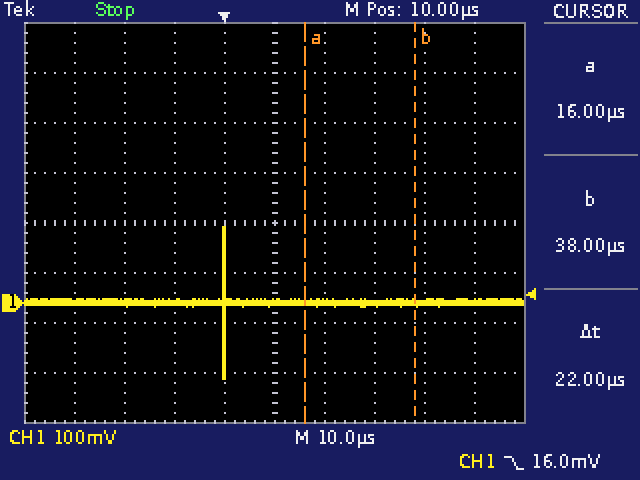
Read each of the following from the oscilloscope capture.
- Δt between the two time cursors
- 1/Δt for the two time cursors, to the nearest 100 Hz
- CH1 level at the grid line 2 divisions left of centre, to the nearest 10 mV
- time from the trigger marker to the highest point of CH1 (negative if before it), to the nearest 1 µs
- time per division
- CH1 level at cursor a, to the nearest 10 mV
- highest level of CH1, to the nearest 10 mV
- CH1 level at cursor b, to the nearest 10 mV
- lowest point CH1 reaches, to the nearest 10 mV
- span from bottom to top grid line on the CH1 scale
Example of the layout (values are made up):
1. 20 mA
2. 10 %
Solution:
1. 22 µs
2. 45.5 kHz
3. 0 mV
4. 0 µs
5. 10 µs
6. 0 mV
7. 150 mV
8. 0 mV
9. -150 mV
10. 800 mV
